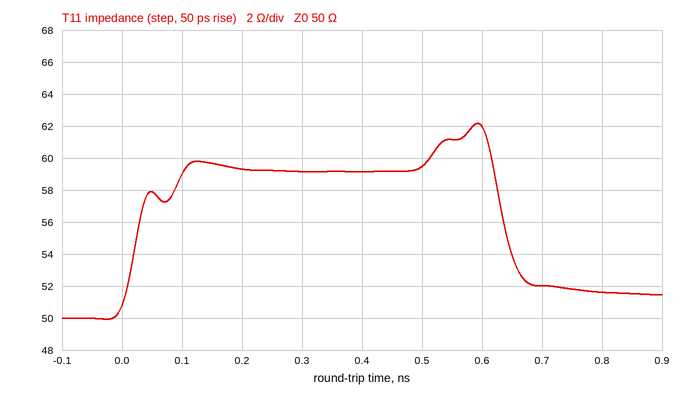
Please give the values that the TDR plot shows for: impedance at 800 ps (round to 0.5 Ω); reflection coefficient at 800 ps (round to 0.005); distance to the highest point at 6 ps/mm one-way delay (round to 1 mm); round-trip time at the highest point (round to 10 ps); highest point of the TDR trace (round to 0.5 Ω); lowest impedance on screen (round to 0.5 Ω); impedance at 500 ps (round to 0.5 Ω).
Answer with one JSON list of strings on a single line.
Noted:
["51.5 Ω", "+0.015", "49 mm", "590 ps", "62.0 Ω", "50.0 Ω", "59.5 Ω"]
